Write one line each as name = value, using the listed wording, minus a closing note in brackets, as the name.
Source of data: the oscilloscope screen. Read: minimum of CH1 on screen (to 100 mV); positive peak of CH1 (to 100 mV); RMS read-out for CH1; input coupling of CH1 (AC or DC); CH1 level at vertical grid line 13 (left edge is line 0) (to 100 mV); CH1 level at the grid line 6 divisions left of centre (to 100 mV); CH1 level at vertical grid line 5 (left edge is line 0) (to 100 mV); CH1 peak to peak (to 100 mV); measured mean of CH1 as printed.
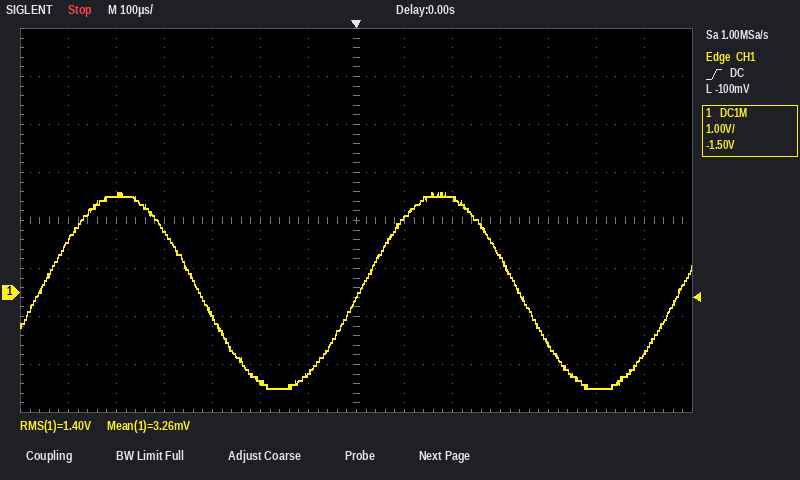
minimum of CH1 on screen = -2.0 V
positive peak of CH1 = 2.1 V
RMS read-out for CH1 = 1.40 V
input coupling of CH1 = DC
CH1 level at vertical grid line 13 (left edge is line 0) = -1.3 V
CH1 level at the grid line 6 divisions left of centre = 1.1 V
CH1 level at vertical grid line 5 (left edge is line 0) = -1.9 V
CH1 peak to peak = 4.1 V
measured mean of CH1 as printed = 3.26 mV
